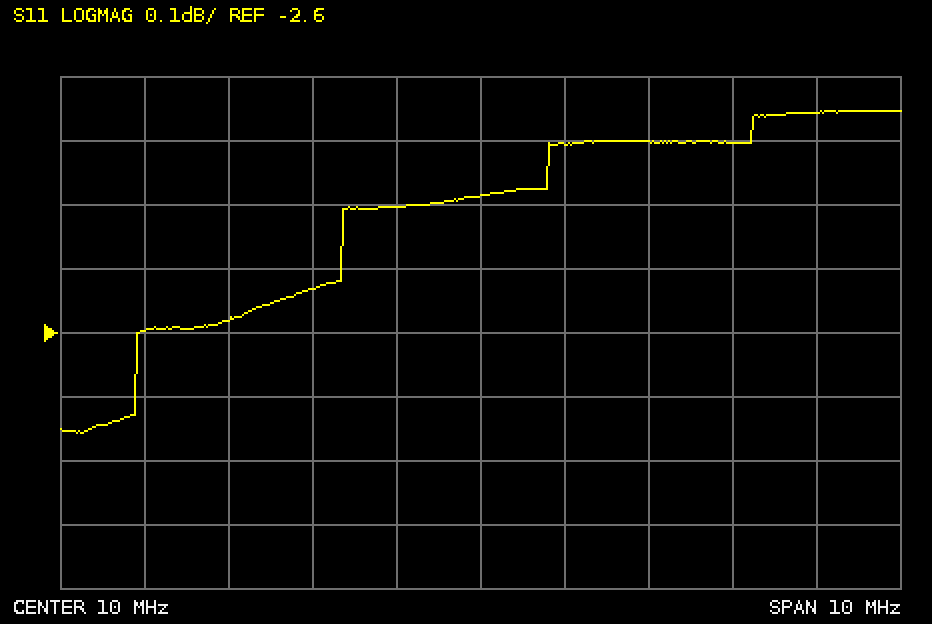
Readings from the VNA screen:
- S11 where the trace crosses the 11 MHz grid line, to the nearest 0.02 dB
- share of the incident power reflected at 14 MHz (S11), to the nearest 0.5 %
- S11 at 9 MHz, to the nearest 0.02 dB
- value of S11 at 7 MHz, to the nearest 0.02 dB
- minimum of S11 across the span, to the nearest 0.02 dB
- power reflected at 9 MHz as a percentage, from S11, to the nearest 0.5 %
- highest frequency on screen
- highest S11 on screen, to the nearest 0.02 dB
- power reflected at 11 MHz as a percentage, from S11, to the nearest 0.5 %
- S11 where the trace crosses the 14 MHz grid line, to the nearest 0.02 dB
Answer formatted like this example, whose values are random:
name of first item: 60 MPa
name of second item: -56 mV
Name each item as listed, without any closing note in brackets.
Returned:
S11 where the trace crosses the 11 MHz grid line, to the nearest 0.02 dB: -2.30 dB
share of the incident power reflected at 14 MHz (S11), to the nearest 0.5 %: 59.5 %
S11 at 9 MHz, to the nearest 0.02 dB: -2.40 dB
value of S11 at 7 MHz, to the nearest 0.02 dB: -2.58 dB
minimum of S11 across the span, to the nearest 0.02 dB: -2.76 dB
power reflected at 9 MHz as a percentage, from S11, to the nearest 0.5 %: 57.5 %
highest frequency on screen: 15 MHz
highest S11 on screen, to the nearest 0.02 dB: -2.26 dB
power reflected at 11 MHz as a percentage, from S11, to the nearest 0.5 %: 59.0 %
S11 where the trace crosses the 14 MHz grid line, to the nearest 0.02 dB: -2.26 dB
